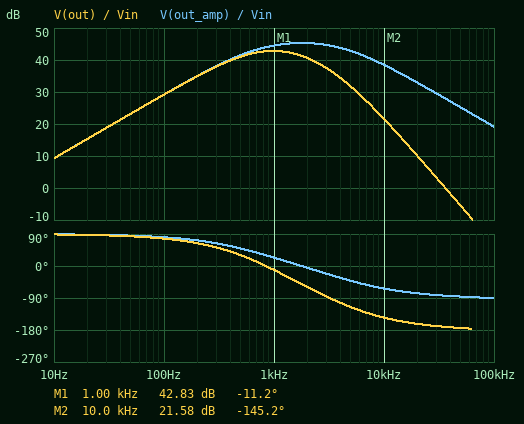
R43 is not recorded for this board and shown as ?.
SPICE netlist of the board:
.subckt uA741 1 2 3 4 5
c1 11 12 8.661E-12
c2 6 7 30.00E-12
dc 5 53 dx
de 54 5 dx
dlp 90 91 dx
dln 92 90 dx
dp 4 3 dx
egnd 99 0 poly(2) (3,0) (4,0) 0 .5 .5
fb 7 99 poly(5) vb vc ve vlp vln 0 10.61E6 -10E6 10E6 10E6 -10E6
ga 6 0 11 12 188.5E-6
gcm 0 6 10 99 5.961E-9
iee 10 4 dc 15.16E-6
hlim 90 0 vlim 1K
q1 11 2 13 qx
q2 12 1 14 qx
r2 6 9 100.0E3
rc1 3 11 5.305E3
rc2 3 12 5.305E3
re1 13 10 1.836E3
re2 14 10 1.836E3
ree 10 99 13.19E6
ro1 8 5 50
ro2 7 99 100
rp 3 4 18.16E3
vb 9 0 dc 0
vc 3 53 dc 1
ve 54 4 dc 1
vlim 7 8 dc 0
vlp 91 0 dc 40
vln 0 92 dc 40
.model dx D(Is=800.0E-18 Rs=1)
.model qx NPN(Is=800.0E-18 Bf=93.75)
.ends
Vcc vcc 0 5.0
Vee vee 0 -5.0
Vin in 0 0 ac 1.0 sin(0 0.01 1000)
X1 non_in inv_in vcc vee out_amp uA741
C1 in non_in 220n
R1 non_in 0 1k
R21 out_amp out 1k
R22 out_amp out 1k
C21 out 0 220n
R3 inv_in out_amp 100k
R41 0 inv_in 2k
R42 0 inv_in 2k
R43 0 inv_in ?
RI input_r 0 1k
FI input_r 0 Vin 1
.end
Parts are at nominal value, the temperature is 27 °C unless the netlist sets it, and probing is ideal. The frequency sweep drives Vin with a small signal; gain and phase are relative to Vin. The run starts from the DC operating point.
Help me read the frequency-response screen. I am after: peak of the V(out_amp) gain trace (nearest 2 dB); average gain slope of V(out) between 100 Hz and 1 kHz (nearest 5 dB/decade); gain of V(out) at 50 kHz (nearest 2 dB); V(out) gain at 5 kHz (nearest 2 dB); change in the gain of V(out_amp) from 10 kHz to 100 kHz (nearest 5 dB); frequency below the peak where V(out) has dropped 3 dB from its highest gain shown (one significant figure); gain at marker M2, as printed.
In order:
46 dB
15 dB/decade
-6 dB
32 dB
-20 dB
400 Hz
21.58 dB
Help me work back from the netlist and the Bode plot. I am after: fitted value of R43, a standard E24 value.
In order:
910 Ω
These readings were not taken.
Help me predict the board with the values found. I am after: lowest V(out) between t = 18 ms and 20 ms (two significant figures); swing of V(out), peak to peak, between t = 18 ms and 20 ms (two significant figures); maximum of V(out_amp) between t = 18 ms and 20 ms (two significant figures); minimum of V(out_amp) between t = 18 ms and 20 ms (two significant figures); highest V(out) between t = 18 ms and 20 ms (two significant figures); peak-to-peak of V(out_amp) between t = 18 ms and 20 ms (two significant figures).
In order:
-1.4 V
2.8 V
1.7 V
-1.7 V
1.4 V
3.4 V
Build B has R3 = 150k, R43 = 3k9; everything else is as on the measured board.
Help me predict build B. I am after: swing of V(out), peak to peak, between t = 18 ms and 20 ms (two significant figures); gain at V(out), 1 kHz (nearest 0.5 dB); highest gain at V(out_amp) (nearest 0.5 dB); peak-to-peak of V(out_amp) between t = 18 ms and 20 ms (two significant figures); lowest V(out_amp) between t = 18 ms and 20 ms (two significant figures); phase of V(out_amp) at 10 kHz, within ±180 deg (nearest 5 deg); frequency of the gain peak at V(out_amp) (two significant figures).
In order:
2.5 V
42.0 dB
44.5 dB
3.0 V
-1.5 V
-60 deg
1.9 kHz
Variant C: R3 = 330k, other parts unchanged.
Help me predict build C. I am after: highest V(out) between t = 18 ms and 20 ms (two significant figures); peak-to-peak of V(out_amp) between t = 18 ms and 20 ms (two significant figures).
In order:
3.7 V
9.0 V
